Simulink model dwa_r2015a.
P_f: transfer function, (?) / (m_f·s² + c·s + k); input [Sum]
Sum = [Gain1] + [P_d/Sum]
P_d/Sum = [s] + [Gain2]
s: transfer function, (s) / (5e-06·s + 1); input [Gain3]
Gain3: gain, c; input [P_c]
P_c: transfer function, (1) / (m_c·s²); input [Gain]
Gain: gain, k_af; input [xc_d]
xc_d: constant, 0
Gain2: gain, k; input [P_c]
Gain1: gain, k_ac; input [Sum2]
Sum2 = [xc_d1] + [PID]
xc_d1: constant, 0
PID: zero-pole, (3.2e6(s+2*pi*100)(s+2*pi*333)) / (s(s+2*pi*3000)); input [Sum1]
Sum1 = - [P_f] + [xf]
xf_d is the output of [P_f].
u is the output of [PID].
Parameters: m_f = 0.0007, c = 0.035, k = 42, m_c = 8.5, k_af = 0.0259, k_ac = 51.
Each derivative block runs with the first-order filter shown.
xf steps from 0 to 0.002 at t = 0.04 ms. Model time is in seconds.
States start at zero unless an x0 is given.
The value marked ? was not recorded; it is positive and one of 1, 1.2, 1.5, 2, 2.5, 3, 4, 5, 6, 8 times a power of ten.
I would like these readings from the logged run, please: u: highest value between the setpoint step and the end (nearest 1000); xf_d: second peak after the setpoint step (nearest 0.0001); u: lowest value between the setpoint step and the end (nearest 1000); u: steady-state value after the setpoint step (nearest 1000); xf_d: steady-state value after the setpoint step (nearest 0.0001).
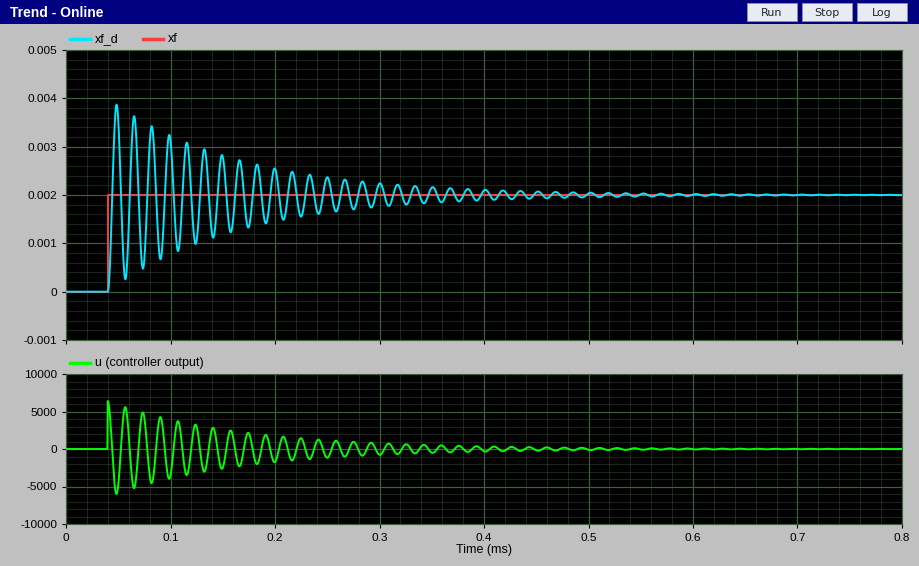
6000
0.0036
-6000
0
0.0020
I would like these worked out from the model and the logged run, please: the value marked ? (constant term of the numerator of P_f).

0.6
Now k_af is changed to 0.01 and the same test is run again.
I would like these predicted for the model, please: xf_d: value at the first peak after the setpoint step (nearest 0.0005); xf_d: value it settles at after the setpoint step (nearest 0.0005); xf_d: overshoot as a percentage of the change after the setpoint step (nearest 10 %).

0.0040
0.0020
90 %
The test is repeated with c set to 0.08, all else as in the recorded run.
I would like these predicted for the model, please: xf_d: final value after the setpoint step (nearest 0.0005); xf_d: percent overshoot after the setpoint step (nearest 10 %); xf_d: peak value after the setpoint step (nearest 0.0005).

0.0020
90 %
0.0040
